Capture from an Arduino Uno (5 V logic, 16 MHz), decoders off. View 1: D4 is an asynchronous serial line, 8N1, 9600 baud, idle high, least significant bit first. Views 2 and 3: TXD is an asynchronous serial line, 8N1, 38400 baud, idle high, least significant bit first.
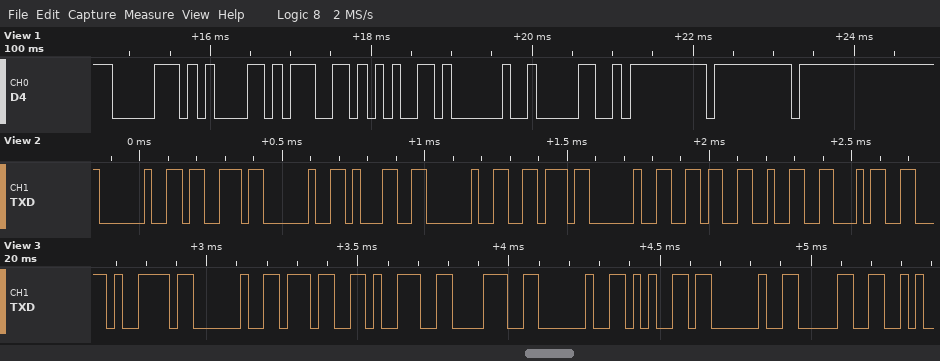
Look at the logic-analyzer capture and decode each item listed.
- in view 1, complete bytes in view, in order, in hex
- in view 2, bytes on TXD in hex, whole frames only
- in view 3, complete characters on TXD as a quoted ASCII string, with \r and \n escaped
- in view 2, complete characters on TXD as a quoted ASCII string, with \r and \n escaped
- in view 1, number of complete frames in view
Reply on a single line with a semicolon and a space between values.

70 61 67 65 20 30 FF FF FF; 20 73 20 31 20 76 20 36 32 34; "y 798 e 0"; " s 1 v 624"; 9
